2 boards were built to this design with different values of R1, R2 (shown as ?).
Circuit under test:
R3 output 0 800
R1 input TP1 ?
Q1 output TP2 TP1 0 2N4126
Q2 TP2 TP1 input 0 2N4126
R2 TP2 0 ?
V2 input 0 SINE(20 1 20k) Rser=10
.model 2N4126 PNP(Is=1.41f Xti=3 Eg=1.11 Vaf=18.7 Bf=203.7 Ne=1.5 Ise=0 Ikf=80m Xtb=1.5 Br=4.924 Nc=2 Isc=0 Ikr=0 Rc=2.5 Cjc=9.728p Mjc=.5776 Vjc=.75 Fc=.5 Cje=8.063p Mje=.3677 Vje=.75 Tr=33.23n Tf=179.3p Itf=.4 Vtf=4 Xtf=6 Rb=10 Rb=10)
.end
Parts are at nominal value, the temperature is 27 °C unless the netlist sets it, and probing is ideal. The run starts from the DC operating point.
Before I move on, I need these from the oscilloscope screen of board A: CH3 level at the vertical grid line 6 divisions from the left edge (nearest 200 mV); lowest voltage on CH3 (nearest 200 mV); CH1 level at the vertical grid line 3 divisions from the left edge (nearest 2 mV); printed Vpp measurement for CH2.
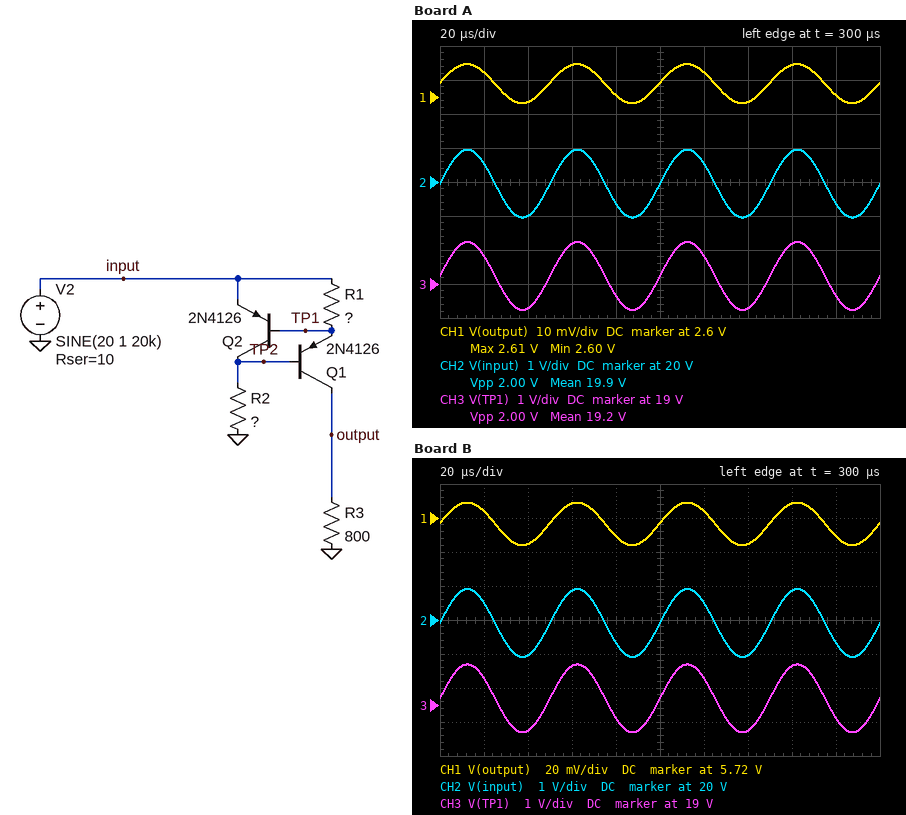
19.8 V
18.2 V
2.610 V
2.00 V
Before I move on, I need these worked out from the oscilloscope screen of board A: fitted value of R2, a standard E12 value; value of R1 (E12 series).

12 kΩ
220 Ω
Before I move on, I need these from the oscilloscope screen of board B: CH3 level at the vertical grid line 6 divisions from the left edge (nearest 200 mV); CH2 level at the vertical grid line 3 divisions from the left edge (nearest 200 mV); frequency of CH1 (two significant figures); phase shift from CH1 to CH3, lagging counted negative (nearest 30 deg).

19.8 V
20.8 V
20 kHz
0 deg
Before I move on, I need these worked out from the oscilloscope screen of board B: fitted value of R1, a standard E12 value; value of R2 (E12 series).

100 Ω
12 kΩ
